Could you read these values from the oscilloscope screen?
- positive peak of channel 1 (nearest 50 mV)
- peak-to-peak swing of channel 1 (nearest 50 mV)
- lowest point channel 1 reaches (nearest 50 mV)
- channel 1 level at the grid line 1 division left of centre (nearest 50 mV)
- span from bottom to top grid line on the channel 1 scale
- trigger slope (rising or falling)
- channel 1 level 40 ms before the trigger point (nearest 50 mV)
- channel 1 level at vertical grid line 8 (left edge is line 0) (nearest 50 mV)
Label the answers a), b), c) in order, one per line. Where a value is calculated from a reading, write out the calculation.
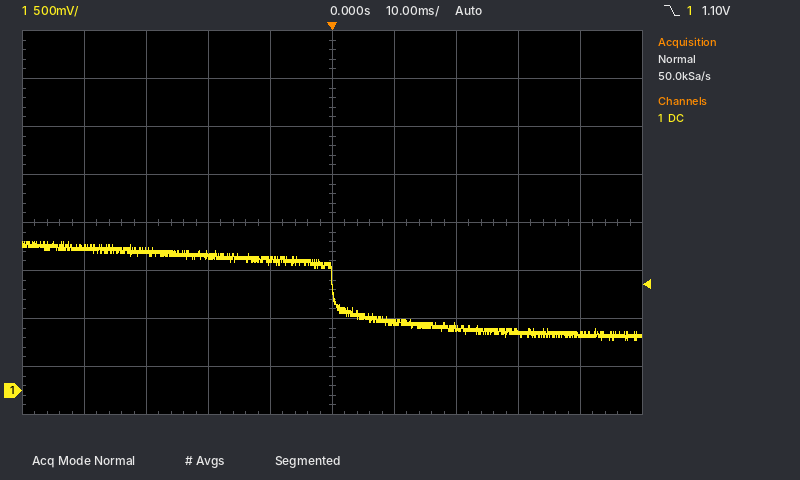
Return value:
a) 1.55 V
b) 1.55 V − (500 mV) = 1.05 V
c) 500 mV
d) 1.35 V
e) 4 V
f) falling
g) 1.50 V
h) 600 mV
